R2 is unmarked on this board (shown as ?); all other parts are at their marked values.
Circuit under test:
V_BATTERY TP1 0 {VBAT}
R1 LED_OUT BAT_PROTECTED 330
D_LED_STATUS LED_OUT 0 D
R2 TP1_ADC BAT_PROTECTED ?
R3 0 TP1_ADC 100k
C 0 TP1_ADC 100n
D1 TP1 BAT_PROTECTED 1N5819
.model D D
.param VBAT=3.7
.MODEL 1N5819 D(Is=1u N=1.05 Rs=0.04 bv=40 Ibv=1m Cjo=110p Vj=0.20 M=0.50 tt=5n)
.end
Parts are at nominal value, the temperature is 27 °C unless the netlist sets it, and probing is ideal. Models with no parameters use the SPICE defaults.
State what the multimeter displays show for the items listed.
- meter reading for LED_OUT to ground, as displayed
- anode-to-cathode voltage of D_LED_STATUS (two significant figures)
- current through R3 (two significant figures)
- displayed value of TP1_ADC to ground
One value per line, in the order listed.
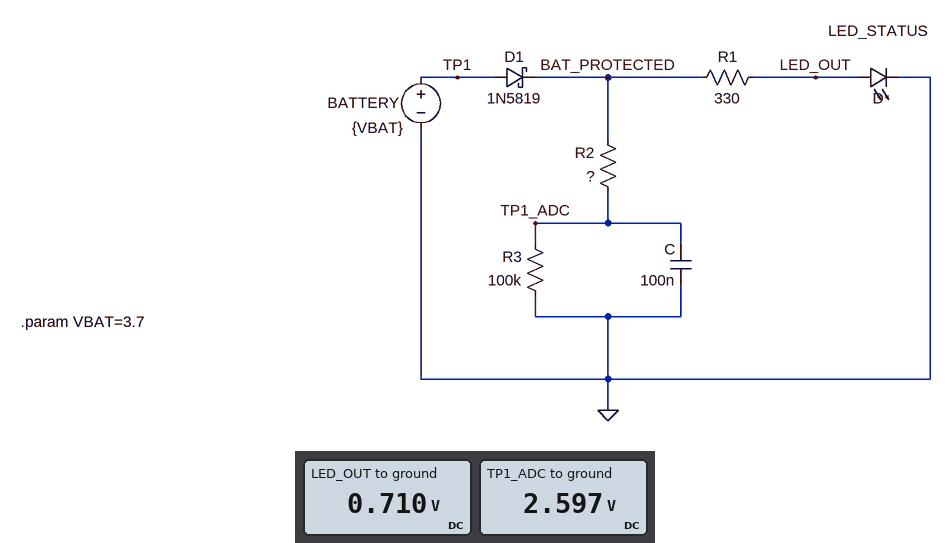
0.710 V
710 mV
26 µA
2.597 V
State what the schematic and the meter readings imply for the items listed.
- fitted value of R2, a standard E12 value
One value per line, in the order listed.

33 kΩ
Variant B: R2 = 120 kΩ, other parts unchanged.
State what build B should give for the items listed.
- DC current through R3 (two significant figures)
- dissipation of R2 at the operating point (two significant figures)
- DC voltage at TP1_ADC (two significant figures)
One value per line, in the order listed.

16 µA
30 µW
1.6 V
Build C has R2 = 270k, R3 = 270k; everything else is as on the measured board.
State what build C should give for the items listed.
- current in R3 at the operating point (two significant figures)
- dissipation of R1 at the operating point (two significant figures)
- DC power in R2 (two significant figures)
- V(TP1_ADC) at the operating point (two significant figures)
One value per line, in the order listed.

6.4 µA
23 mW
11 µW
1.7 V
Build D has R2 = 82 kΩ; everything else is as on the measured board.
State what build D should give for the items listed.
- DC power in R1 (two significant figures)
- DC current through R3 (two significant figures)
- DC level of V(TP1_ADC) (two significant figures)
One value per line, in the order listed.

23 mW
19 µA
1.9 V
